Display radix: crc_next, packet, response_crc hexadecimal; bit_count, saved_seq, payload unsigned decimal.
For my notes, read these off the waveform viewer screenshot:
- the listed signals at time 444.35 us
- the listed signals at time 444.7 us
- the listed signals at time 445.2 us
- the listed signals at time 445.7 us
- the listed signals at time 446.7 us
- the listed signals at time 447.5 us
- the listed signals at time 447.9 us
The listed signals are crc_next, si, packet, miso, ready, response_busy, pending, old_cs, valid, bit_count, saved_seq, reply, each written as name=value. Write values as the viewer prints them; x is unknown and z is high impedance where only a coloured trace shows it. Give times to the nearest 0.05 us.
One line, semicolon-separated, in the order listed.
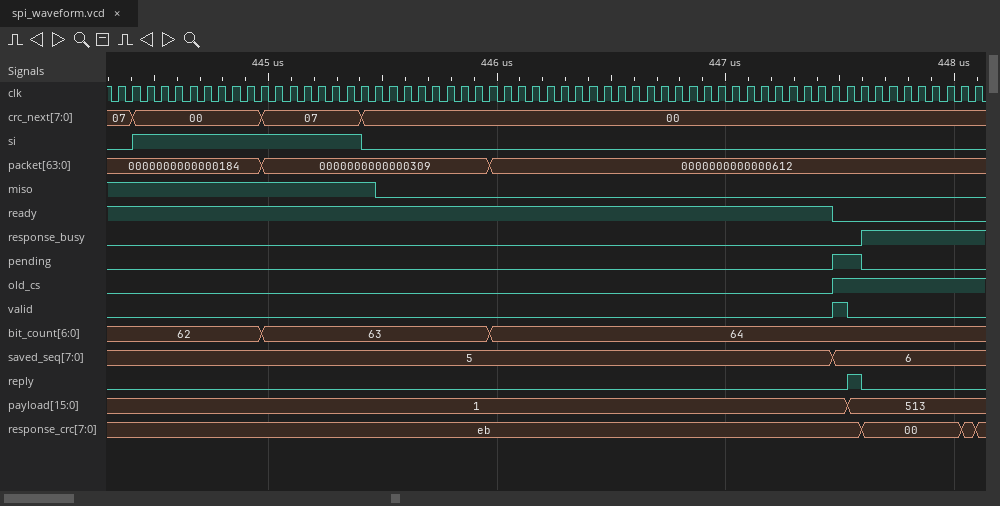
crc_next=07, si=0, packet=0000000000000184, miso=1, ready=1, response_busy=0, pending=0, old_cs=0, valid=0, bit_count=62, saved_seq=5, reply=0; crc_next=00, si=1, packet=0000000000000184, miso=1, ready=1, response_busy=0, pending=0, old_cs=0, valid=0, bit_count=62, saved_seq=5, reply=0; crc_next=07, si=1, packet=0000000000000309, miso=1, ready=1, response_busy=0, pending=0, old_cs=0, valid=0, bit_count=63, saved_seq=5, reply=0; crc_next=00, si=0, packet=0000000000000309, miso=0, ready=1, response_busy=0, pending=0, old_cs=0, valid=0, bit_count=63, saved_seq=5, reply=0; crc_next=00, si=0, packet=0000000000000612, miso=0, ready=1, response_busy=0, pending=0, old_cs=0, valid=0, bit_count=64, saved_seq=5, reply=0; crc_next=00, si=0, packet=0000000000000612, miso=0, ready=0, response_busy=0, pending=1, old_cs=1, valid=1, bit_count=64, saved_seq=6, reply=0; crc_next=00, si=0, packet=0000000000000612, miso=0, ready=0, response_busy=1, pending=0, old_cs=1, valid=0, bit_count=64, saved_seq=6, reply=0
